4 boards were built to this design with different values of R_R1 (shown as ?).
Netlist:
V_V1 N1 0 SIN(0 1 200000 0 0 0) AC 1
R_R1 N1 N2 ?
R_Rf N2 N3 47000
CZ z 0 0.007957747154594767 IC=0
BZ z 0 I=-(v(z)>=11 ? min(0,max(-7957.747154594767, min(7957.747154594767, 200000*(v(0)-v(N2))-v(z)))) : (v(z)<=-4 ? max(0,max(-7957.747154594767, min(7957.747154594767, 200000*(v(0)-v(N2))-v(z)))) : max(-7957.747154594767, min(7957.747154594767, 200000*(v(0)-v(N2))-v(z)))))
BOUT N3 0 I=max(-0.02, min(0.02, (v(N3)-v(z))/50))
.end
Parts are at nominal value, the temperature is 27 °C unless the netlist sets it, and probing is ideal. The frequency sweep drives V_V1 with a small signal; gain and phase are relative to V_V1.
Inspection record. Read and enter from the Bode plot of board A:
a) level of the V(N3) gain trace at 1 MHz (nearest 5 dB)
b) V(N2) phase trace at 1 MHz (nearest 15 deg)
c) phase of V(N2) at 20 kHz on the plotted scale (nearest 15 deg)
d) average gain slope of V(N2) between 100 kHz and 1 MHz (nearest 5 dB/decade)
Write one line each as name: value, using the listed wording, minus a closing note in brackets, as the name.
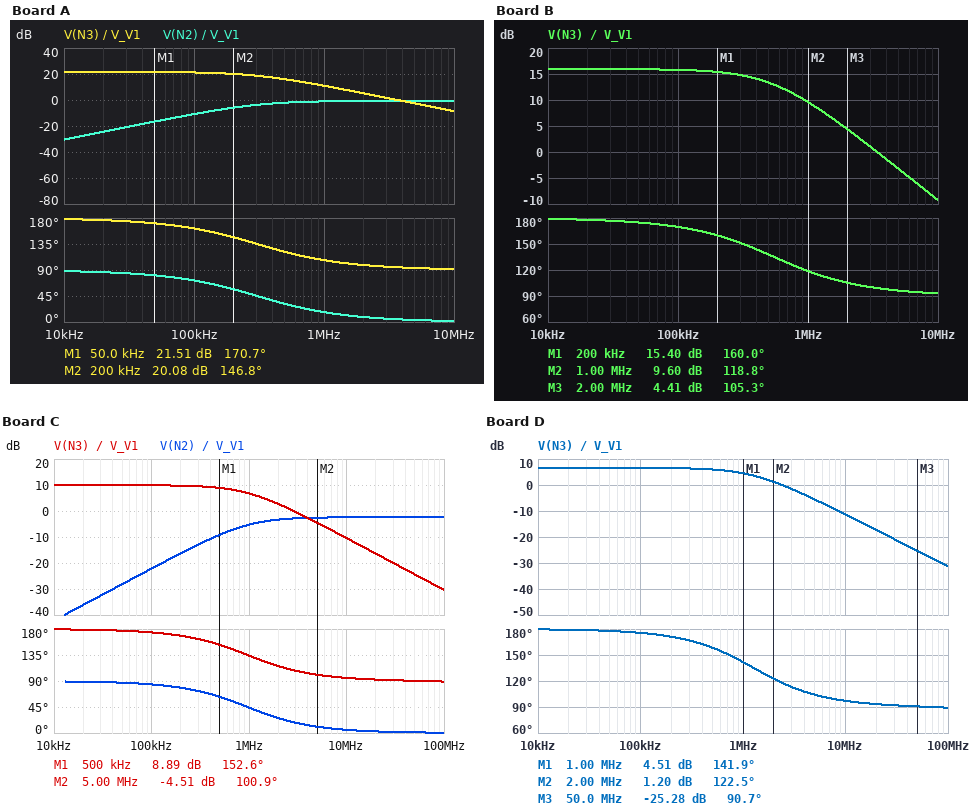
level of the V(N3) gain trace at 1 MHz: 10 dB
V(N2) phase trace at 1 MHz: 15 deg
phase of V(N2) at 20 kHz on the plotted scale: 90 deg
average gain slope of V(N2) between 100 kHz and 1 MHz: 10 dB/decade
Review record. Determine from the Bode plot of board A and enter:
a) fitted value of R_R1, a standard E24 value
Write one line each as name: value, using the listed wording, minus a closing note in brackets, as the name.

fitted value of R_R1, a standard E24 value: 3.9 kΩ
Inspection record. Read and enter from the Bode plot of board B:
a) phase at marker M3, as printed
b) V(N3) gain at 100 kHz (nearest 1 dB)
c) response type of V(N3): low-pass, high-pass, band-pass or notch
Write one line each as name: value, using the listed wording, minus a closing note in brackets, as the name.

phase at marker M3, as printed: 105.3 deg
V(N3) gain at 100 kHz: 16 dB
response type of V(N3): low-pass, high-pass, band-pass or notch: low-pass
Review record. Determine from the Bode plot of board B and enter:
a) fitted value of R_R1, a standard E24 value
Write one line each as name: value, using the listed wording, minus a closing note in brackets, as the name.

fitted value of R_R1, a standard E24 value: 7.5 kΩ
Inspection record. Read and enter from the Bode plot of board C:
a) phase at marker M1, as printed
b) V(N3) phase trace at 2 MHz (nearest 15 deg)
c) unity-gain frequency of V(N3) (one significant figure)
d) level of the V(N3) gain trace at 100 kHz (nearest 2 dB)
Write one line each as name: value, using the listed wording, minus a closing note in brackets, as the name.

phase at marker M1, as printed: 152.6 deg
V(N3) phase trace at 2 MHz: 120 deg
unity-gain frequency of V(N3): 3 MHz
level of the V(N3) gain trace at 100 kHz: 10 dB
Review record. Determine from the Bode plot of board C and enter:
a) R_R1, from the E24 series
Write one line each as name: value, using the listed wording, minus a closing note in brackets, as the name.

R_R1, from the E24 series: 15 kΩ
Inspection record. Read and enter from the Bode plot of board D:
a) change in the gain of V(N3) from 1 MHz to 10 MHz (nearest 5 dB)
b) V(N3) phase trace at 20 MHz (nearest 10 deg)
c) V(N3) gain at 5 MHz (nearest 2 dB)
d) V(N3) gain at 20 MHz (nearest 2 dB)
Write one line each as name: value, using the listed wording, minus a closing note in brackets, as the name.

change in the gain of V(N3) from 1 MHz to 10 MHz: -15 dB
V(N3) phase trace at 20 MHz: 90 deg
V(N3) gain at 5 MHz: -6 dB
V(N3) gain at 20 MHz: -18 dB
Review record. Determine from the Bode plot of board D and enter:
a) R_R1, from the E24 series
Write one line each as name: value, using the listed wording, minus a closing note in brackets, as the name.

R_R1, from the E24 series: 22 kΩ
